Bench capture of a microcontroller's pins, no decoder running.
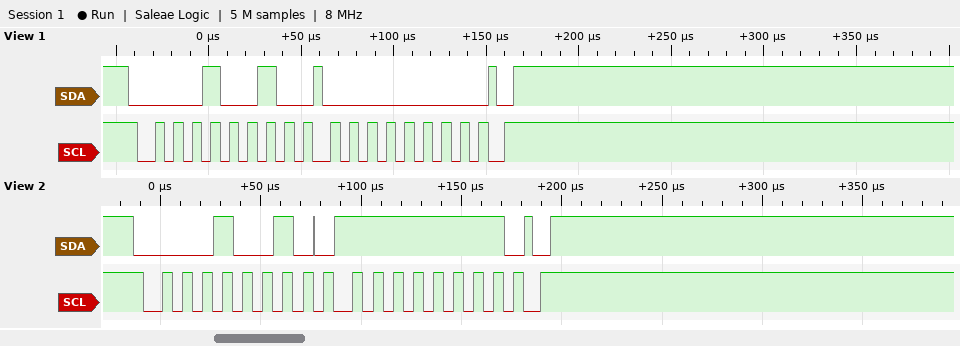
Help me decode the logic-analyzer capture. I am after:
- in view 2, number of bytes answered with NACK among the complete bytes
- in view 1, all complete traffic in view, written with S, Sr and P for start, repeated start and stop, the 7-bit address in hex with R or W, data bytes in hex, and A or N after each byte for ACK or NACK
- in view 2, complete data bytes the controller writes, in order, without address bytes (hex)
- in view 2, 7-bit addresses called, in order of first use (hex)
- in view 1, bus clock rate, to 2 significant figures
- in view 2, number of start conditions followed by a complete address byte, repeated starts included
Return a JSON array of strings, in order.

["0", "S 09W A 00 A P", "FF", "0x09", "100 kHz", "1"]
